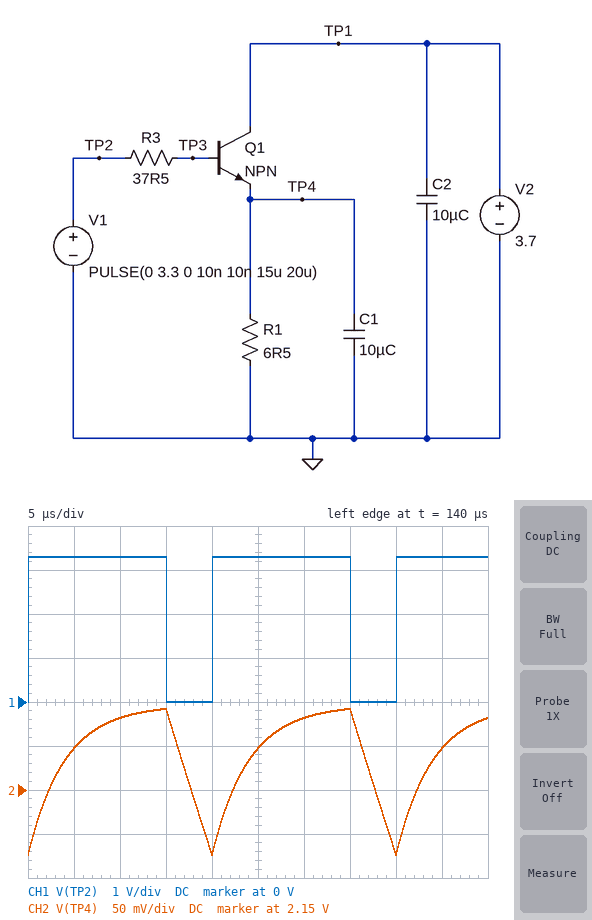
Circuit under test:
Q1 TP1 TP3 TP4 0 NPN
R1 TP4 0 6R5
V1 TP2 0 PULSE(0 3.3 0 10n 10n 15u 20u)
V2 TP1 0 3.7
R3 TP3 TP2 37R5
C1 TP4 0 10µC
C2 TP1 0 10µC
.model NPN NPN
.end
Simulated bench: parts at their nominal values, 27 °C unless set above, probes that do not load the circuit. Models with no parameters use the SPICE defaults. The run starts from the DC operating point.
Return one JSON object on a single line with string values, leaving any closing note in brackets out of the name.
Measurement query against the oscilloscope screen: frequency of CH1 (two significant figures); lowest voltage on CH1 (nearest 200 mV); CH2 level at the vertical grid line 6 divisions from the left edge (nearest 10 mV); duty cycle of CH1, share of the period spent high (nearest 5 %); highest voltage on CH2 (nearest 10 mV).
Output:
{"frequency of CH1": "50 kHz", "lowest voltage on CH1": "0 V", "CH2 level at the vertical grid line 6 divisions from the left edge": "2.23 V", "duty cycle of CH1, share of the period spent high": "75 %", "highest voltage on CH2": "2.24 V"}
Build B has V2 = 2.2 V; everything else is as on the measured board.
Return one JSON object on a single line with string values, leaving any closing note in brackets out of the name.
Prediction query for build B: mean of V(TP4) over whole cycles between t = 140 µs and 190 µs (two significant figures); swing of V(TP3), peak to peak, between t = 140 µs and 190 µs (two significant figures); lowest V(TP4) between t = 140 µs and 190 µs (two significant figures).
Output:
{"mean of V(TP4) over whole cycles between t = 140 µs and 190 µs": "2.1 V", "swing of V(TP3), peak to peak, between t = 140 µs and 190 µs": "3.0 V", "lowest V(TP4) between t = 140 µs and 190 µs": "1.9 V"}
